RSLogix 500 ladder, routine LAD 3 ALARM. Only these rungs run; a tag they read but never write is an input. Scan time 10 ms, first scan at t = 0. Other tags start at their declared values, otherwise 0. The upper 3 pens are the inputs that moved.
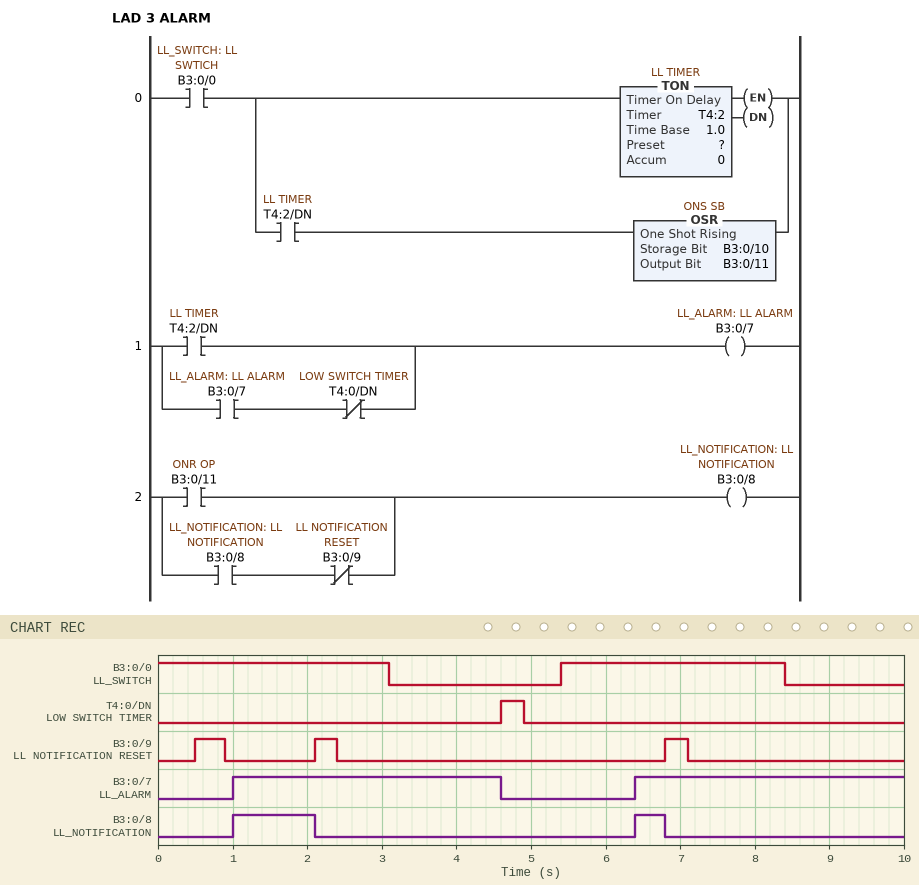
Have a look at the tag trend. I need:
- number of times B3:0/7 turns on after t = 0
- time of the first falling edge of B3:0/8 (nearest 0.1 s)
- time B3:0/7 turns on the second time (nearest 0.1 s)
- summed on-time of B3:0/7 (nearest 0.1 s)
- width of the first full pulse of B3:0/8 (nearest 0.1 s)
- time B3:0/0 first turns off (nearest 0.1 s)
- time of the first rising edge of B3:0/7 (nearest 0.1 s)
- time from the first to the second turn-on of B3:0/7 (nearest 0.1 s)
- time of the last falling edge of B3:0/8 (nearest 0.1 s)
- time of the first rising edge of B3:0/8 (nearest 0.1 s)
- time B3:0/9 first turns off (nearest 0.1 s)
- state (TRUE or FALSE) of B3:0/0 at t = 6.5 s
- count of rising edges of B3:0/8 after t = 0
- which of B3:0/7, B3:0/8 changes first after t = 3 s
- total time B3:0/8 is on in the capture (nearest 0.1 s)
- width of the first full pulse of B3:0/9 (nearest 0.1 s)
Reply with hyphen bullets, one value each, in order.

- 2
- 2.1 s
- 6.4 s
- 7.2 s
- 1.1 s
- 3.1 s
- 1.0 s
- 5.4 s
- 6.8 s
- 1.0 s
- 0.9 s
- TRUE
- 2
- B3:0/7
- 1.5 s
- 0.4 s
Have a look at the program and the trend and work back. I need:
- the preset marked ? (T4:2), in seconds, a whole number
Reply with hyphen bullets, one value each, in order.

- 1 s
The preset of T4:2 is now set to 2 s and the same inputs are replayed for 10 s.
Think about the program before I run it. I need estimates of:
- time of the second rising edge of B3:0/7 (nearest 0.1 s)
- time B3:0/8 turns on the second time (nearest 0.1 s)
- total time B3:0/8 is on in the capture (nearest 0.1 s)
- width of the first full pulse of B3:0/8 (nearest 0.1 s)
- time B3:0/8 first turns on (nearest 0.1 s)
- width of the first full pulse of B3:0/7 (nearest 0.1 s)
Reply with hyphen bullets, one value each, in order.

- 7.4 s
- 7.4 s
- 2.7 s
- 0.1 s
- 2.0 s
- 2.6 s
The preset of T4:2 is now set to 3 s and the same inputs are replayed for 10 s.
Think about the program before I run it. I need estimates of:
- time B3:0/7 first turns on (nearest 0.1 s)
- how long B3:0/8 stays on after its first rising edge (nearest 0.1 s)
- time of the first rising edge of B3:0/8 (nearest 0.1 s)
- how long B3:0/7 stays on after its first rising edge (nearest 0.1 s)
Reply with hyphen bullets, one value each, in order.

- 3.0 s
- 3.8 s
- 3.0 s
- 1.6 s
